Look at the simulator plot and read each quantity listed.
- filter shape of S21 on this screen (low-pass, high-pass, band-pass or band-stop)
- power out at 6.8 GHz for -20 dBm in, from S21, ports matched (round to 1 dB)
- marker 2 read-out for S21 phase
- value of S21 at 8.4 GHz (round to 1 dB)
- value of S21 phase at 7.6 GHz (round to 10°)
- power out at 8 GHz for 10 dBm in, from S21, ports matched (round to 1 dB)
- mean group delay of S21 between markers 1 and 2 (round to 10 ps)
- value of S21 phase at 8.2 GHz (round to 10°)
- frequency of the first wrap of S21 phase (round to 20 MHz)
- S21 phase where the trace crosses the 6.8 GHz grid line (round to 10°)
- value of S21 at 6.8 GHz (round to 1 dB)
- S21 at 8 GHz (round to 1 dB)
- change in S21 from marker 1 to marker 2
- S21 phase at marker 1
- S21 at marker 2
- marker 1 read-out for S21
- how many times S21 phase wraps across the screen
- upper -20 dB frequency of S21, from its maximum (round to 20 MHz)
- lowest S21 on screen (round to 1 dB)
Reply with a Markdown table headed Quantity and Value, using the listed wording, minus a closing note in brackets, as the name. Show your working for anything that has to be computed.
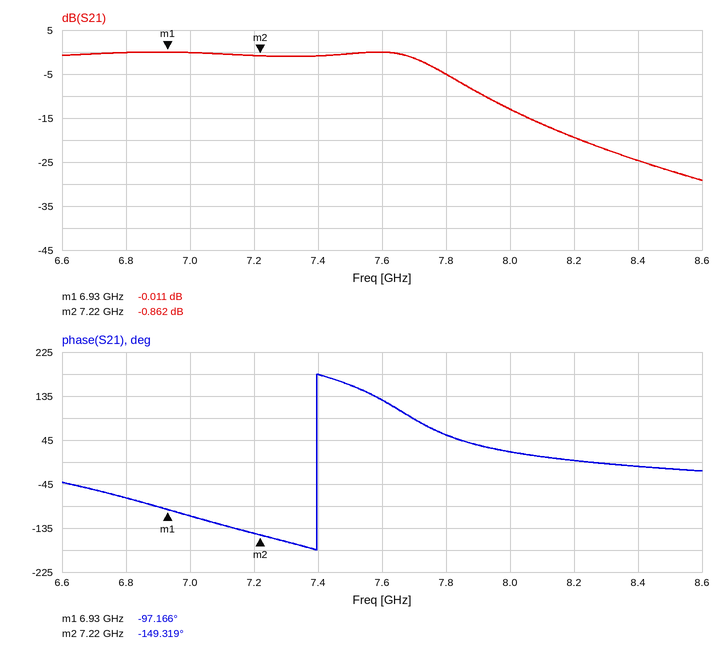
| Quantity | Value |
|---|---|
| filter shape of S21 on this screen | low-pass |
| power out at 6.8 GHz for -20 dBm in, from S21, ports matched | -20 dBm + (0 dB) = -20 dBm |
| marker 2 read-out for S21 phase | -149.319° |
| value of S21 at 8.4 GHz | -25 dB |
| value of S21 phase at 7.6 GHz | 130° |
| power out at 8 GHz for 10 dBm in, from S21, ports matched | 10 dBm + (-13 dB) = -3 dBm |
| mean group delay of S21 between markers 1 and 2 | −(-149.319° − (-97.166°))/(360° × 290 MHz) ≈ 500 ps |
| value of S21 phase at 8.2 GHz | 0° |
| frequency of the first wrap of S21 phase | 7.40 GHz |
| S21 phase where the trace crosses the 6.8 GHz grid line | -70° |
| value of S21 at 6.8 GHz | 0 dB |
| S21 at 8 GHz | -13 dB |
| change in S21 from marker 1 to marker 2 | -0.862 − (-0.011) = -0.851 dB |
| S21 phase at marker 1 | -97.166° |
| S21 at marker 2 | -0.862 dB |
| marker 1 read-out for S21 | -0.011 dB |
| how many times S21 phase wraps across the screen | 1 |
| upper -20 dB frequency of S21, from its maximum | 8.22 GHz |
| lowest S21 on screen | -29 dB |
